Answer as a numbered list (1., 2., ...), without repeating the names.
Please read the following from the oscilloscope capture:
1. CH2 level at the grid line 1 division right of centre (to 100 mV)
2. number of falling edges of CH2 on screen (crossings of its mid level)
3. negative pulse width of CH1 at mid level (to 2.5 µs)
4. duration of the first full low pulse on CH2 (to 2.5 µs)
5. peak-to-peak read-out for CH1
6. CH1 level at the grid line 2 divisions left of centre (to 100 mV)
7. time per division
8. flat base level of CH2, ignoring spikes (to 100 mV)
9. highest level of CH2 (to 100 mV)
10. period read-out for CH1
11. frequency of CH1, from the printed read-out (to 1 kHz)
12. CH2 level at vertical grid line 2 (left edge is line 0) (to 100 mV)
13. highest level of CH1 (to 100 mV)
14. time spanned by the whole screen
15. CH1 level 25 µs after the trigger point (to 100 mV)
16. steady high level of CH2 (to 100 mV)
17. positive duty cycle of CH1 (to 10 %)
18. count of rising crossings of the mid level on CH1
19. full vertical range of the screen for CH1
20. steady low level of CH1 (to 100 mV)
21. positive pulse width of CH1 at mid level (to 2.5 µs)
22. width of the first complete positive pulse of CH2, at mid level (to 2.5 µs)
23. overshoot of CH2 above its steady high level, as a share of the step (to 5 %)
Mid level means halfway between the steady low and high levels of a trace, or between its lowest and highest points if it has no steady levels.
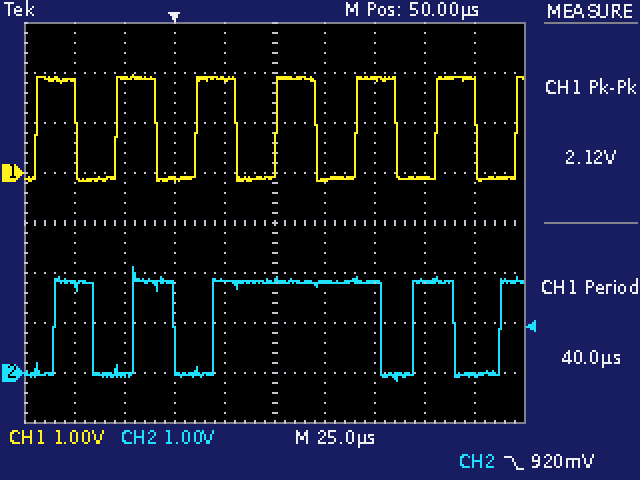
1. 1.8 V
2. 4
3. 20.0 µs
4. 20.0 µs
5. 2.12 V
6. -100 mV
7. 25 µs
8. 0.0 V
9. 2.1 V
10. 40.0 µs
11. 25 kHz
12. 0.0 V
13. 2.0 V
14. 250 µs
15. 1.9 V
16. 1.8 V
17. 50 %
18. 7
19. 8 V
20. -100 mV
21. 20.0 µs
22. 20.0 µs
23. 15 %
